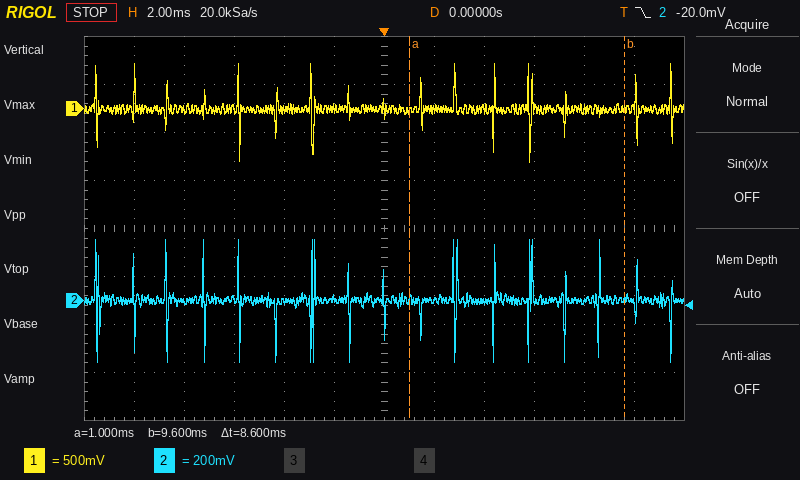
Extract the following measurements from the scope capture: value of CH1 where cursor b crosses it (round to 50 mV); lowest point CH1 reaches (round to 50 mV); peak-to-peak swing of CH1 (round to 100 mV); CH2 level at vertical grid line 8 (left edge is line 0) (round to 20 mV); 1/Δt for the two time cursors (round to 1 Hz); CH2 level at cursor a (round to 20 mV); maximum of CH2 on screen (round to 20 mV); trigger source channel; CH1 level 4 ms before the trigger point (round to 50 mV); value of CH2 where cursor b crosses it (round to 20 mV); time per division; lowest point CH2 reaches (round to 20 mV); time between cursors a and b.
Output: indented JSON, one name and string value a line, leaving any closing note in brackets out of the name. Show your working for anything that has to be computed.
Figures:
{
  "value of CH1 where cursor b crosses it": "0 mV",
  "lowest point CH1 reaches": "-550 mV",
  "peak-to-peak swing of CH1": "1.00 V",
  "CH2 level at vertical grid line 8 (left edge is line 0)": "0 mV",
  "1/Δt for the two time cursors": "1 / 8.6 ms ≈ 116 Hz",
  "CH2 level at cursor a": "0 mV",
  "maximum of CH2 on screen": "260 mV",
  "trigger source channel": "CH2",
  "CH1 level 4 ms before the trigger point": "0 mV",
  "value of CH2 where cursor b crosses it": "20 mV",
  "time per division": "2 ms",
  "lowest point CH2 reaches": "-260 mV",
  "time between cursors a and b": "8.6 ms"
}
